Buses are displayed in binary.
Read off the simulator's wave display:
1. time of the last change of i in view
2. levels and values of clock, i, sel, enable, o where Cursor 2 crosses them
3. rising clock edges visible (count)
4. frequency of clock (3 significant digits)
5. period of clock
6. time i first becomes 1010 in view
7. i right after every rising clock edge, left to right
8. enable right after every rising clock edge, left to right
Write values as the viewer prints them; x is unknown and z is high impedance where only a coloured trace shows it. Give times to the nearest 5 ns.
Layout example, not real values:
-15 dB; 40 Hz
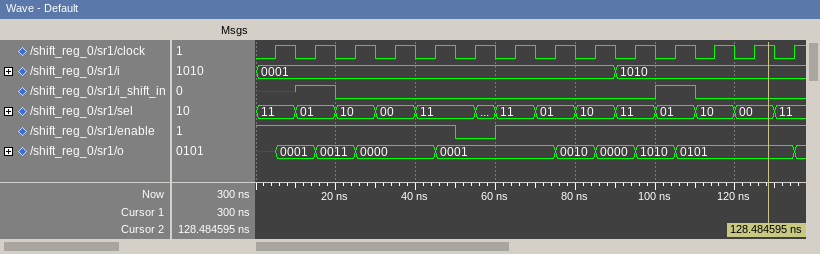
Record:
90 ns; clock=1, i=1010, sel=00, enable=1, o=0101; 14; 100 MHz; 10 ns; 90 ns; 0001, 0001, 0001, 0001, 0001, 0001, 0001, 0001, 0001, 1010, 1010, 1010, 1010, 1010; 1 1 1 1 1 0 1 1 1 1 1 1 1 1
